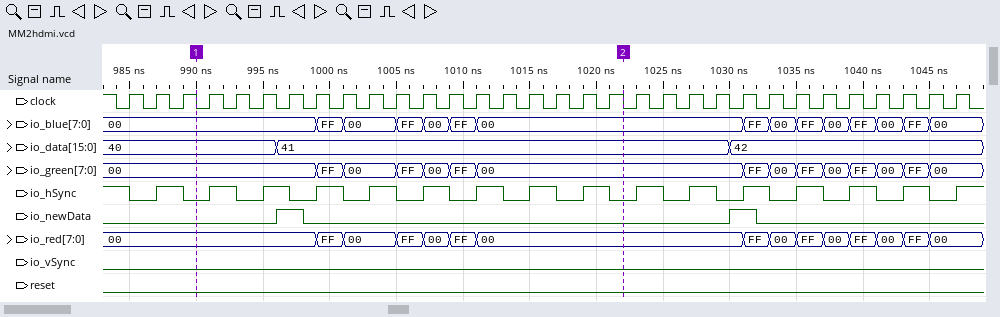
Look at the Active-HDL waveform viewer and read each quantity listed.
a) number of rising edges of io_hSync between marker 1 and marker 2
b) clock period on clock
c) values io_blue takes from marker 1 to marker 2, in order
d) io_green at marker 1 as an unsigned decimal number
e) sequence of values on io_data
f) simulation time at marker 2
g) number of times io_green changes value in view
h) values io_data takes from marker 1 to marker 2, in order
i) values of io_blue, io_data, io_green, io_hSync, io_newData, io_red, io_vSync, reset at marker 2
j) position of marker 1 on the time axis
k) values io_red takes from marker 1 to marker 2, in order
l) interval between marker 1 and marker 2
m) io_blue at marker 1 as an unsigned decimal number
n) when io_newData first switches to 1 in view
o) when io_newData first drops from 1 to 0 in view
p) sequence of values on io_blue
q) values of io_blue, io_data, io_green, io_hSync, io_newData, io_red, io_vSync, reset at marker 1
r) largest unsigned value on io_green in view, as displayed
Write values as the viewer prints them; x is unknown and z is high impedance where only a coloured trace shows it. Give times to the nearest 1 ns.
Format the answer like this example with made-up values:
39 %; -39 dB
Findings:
8; 2 ns; 00, FF, 00, FF, 00, FF, 00; 0; 40, 41, 42; 1022 ns; 14; 40, 41; io_blue=00, io_data=41, io_green=00, io_hSync=0, io_newData=0, io_red=00, io_vSync=0, reset=0; 990 ns; 00, FF, 00, FF, 00, FF, 00; 32 ns; 0; 996 ns; 998 ns; 00, FF, 00, FF, 00, FF, 00, FF, 00, FF, 00, FF, 00, FF, 00; io_blue=00, io_data=40, io_green=00, io_hSync=0, io_newData=0, io_red=00, io_vSync=0, reset=0; FF
